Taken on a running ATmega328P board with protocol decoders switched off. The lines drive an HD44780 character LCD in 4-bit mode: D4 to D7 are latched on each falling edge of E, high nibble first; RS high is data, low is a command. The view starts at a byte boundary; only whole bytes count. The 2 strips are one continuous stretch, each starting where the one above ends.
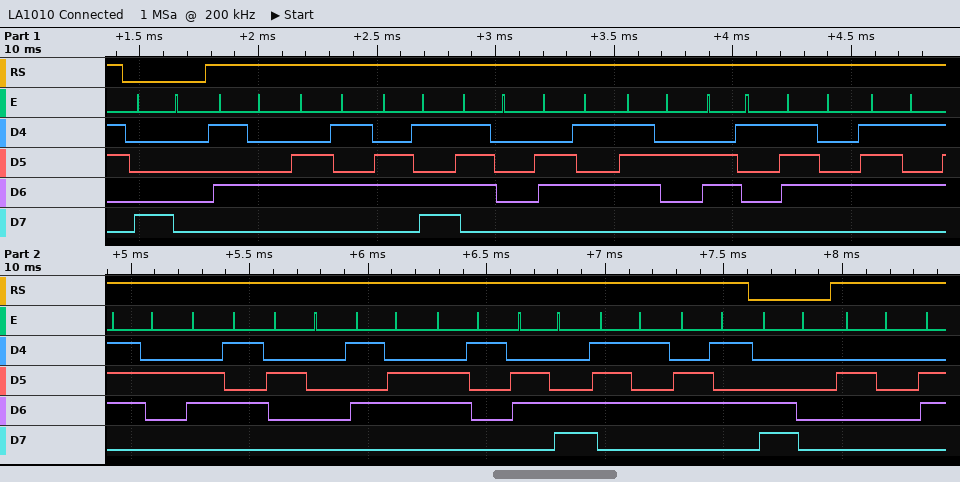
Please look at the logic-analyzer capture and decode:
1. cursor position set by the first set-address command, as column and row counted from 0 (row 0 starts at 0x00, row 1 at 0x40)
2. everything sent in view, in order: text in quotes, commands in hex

column 0, row 0
0x80 "Temperature Value" 0xC0 " "
